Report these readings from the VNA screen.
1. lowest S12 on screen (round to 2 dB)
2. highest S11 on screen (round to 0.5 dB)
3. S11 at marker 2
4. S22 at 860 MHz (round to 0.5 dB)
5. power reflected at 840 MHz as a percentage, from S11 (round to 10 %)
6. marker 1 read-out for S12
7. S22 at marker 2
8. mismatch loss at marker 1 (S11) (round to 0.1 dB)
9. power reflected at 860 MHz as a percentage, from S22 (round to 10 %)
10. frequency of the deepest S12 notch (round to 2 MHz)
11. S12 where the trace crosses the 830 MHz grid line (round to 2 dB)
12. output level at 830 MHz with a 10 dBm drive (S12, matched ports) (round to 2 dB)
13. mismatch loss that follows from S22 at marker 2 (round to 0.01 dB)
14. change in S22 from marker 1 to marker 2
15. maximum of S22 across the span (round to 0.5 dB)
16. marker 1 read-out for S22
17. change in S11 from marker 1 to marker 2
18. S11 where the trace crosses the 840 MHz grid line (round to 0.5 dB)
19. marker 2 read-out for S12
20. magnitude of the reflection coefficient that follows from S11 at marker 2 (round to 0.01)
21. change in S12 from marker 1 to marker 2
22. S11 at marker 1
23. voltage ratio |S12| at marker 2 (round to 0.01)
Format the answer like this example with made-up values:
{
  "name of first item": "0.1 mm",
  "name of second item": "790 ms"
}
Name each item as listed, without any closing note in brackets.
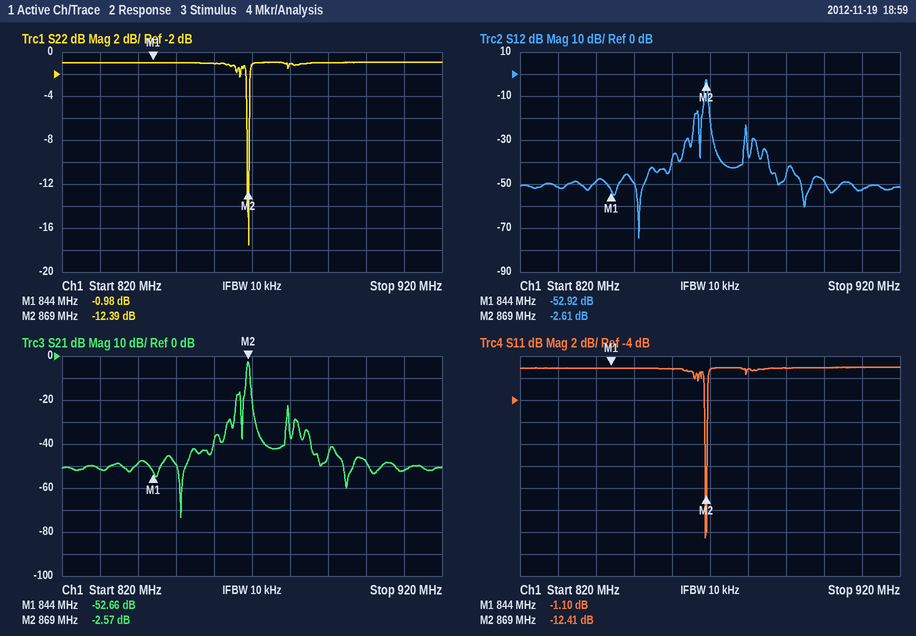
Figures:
{
  "lowest S12 on screen": "-74 dB",
  "highest S11 on screen": "-1.0 dB",
  "S11 at marker 2": "-12.41 dB",
  "S22 at 860 MHz": "-1.0 dB",
  "power reflected at 840 MHz as a percentage, from S11": "80 %",
  "marker 1 read-out for S12": "-52.92 dB",
  "S22 at marker 2": "-12.39 dB",
  "mismatch loss at marker 1 (S11)": "6.5 dB",
  "power reflected at 860 MHz as a percentage, from S22": "80 %",
  "frequency of the deepest S12 notch": "852 MHz",
  "S12 where the trace crosses the 830 MHz grid line": "-52 dB",
  "output level at 830 MHz with a 10 dBm drive (S12, matched ports)": "-42 dBm",
  "mismatch loss that follows from S22 at marker 2": "0.26 dB",
  "change in S22 from marker 1 to marker 2": "-11.41 dB",
  "maximum of S22 across the span": "-1.0 dB",
  "marker 1 read-out for S22": "-0.98 dB",
  "change in S11 from marker 1 to marker 2": "-11.31 dB",
  "S11 where the trace crosses the 840 MHz grid line": "-1.0 dB",
  "marker 2 read-out for S12": "-2.61 dB",
  "magnitude of the reflection coefficient that follows from S11 at marker 2": "0.24",
  "change in S12 from marker 1 to marker 2": "50.31 dB",
  "S11 at marker 1": "-1.10 dB",
  "voltage ratio |S12| at marker 2": "0.74"
}
